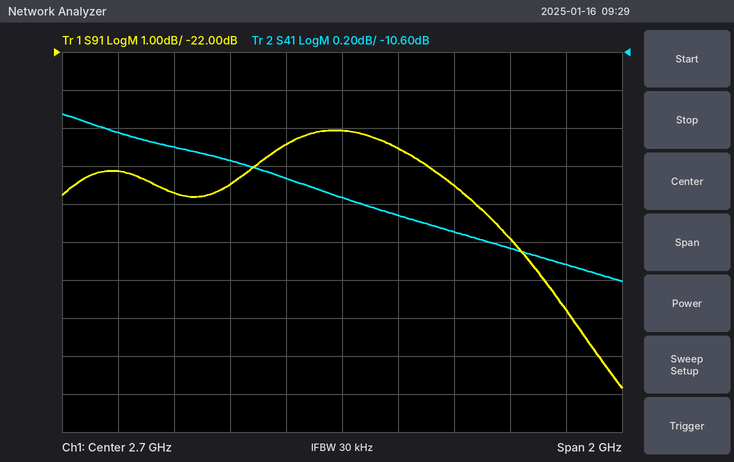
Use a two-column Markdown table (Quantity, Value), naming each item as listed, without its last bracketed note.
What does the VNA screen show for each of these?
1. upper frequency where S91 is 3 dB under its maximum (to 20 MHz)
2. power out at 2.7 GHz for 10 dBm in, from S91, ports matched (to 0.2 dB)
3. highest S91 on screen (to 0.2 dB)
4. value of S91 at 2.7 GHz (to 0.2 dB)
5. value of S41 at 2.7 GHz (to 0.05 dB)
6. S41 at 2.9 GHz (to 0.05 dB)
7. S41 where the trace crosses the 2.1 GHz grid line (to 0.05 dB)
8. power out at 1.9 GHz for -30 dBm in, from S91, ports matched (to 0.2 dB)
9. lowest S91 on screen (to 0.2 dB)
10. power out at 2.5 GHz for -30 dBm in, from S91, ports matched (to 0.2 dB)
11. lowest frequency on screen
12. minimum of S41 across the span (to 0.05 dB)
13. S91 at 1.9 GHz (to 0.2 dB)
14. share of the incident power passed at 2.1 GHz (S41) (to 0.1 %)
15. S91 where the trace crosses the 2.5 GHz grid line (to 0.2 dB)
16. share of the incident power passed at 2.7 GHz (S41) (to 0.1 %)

| Quantity | Value |
|---|---|
| upper frequency where S91 is 3 dB under its maximum | 3.32 GHz |
| power out at 2.7 GHz for 10 dBm in, from S91, ports matched | -14.0 dBm |
| highest S91 on screen | -24.0 dB |
| value of S91 at 2.7 GHz | -24.0 dB |
| value of S41 at 2.7 GHz | -11.35 dB |
| S41 at 2.9 GHz | -11.45 dB |
| S41 where the trace crosses the 2.1 GHz grid line | -11.10 dB |
| power out at 1.9 GHz for -30 dBm in, from S91, ports matched | -55.2 dBm |
| lowest S91 on screen | -30.8 dB |
| power out at 2.5 GHz for -30 dBm in, from S91, ports matched | -54.4 dBm |
| lowest frequency on screen | 1.7 GHz |
| minimum of S41 across the span | -11.80 dB |
| S91 at 1.9 GHz | -25.2 dB |
| share of the incident power passed at 2.1 GHz (S41) | 7.8 % |
| S91 where the trace crosses the 2.5 GHz grid line | -24.4 dB |
| share of the incident power passed at 2.7 GHz (S41) | 7.3 % |
